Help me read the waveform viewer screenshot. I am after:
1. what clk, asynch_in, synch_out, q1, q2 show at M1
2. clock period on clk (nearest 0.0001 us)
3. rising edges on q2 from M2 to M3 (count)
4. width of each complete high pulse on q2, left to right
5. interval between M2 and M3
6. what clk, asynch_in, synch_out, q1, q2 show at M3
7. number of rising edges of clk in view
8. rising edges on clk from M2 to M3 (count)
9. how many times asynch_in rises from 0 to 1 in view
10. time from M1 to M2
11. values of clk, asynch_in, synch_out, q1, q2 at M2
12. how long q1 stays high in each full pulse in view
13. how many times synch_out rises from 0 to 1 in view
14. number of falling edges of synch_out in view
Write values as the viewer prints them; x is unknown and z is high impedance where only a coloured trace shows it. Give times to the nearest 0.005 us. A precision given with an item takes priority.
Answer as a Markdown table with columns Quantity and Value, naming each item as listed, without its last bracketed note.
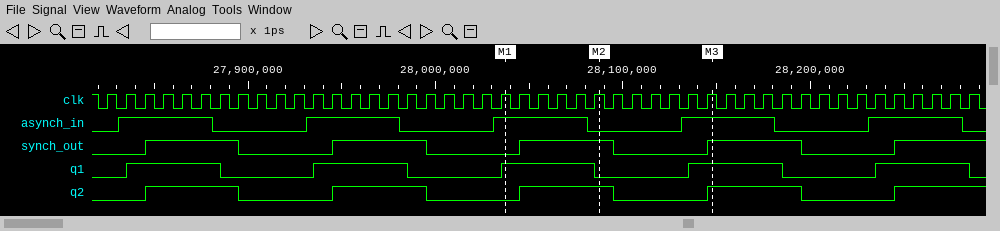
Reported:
| Quantity | Value |
|---|---|
| what clk, asynch_in, synch_out, q1, q2 show at M1 | clk=1, asynch_in=1, synch_out=0, q1=1, q2=0 |
| clock period on clk | 0.01 us |
| rising edges on q2 from M2 to M3 | 1 |
| width of each complete high pulse on q2, left to right | 0.05 us, 0.05 us, 0.05 us, 0.05 us |
| interval between M2 and M3 | 0.06 us |
| what clk, asynch_in, synch_out, q1, q2 show at M3 | clk=1, asynch_in=1, synch_out=1, q1=1, q2=1 |
| number of rising edges of clk in view | 47 |
| rising edges on clk from M2 to M3 | 6 |
| how many times asynch_in rises from 0 to 1 in view | 5 |
| time from M1 to M2 | 0.05 us |
| values of clk, asynch_in, synch_out, q1, q2 at M2 | clk=1, asynch_in=0, synch_out=1, q1=0, q2=1 |
| how long q1 stays high in each full pulse in view | 0.05 us, 0.05 us, 0.05 us, 0.05 us, 0.05 us |
| how many times synch_out rises from 0 to 1 in view | 5 |
| number of falling edges of synch_out in view | 4 |
